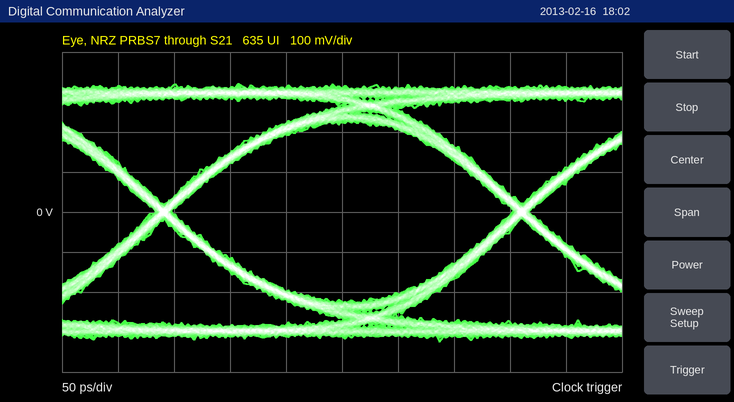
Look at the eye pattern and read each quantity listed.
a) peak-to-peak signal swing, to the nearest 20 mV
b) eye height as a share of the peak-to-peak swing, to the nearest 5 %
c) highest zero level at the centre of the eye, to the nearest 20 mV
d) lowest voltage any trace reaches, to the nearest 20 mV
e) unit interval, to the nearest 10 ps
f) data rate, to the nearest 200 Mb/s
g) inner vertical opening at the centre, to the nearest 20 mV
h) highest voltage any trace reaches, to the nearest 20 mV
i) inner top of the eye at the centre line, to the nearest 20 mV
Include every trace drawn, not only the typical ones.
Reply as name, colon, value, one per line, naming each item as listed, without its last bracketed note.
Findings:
peak-to-peak signal swing, to the nearest 20 mV: 640 mV
eye height as a share of the peak-to-peak swing, to the nearest 5 %: 70 %
highest zero level at the centre of the eye, to the nearest 20 mV: -220 mV
lowest voltage any trace reaches, to the nearest 20 mV: -320 mV
unit interval, to the nearest 10 ps: 320 ps
data rate, to the nearest 200 Mb/s: 3.2 Gb/s
inner vertical opening at the centre, to the nearest 20 mV: 440 mV
highest voltage any trace reaches, to the nearest 20 mV: 320 mV
inner top of the eye at the centre line, to the nearest 20 mV: 220 mV
